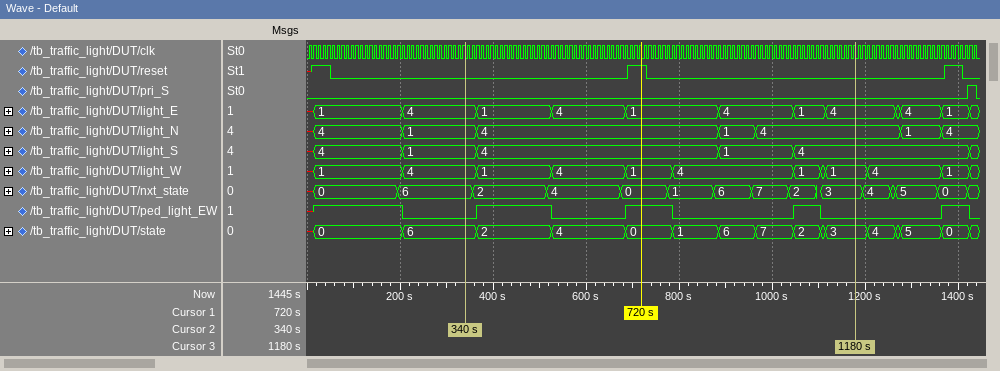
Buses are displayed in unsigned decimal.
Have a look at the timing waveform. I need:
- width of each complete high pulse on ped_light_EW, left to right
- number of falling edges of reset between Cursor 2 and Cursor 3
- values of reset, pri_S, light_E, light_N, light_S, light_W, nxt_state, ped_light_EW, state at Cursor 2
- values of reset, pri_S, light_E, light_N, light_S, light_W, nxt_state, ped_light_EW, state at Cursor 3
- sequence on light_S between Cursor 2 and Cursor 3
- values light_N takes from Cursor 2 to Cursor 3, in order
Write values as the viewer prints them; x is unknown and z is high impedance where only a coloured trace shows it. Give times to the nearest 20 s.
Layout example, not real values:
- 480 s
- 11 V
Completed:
- 160 s, 100 s, 60 s, 60 s
- 1
- reset=0, pri_S=0, light_E=4, light_N=1, light_S=1, light_W=4, nxt_state=6, ped_light_EW=0, state=6
- reset=0, pri_S=0, light_E=4, light_N=4, light_S=4, light_W=1, nxt_state=3, ped_light_EW=0, state=3
- 1, 4, 1, 4
- 1, 4, 1, 4
